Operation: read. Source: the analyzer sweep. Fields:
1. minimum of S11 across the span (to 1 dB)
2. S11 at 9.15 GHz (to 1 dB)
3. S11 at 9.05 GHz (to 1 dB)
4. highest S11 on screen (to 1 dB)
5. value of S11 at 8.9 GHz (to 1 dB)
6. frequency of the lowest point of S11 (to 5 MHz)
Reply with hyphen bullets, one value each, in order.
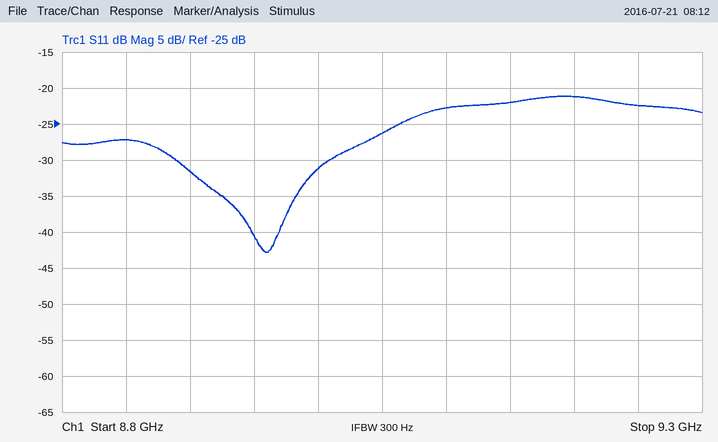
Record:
- -43 dB
- -22 dB
- -26 dB
- -21 dB
- -32 dB
- 8.960 GHz
